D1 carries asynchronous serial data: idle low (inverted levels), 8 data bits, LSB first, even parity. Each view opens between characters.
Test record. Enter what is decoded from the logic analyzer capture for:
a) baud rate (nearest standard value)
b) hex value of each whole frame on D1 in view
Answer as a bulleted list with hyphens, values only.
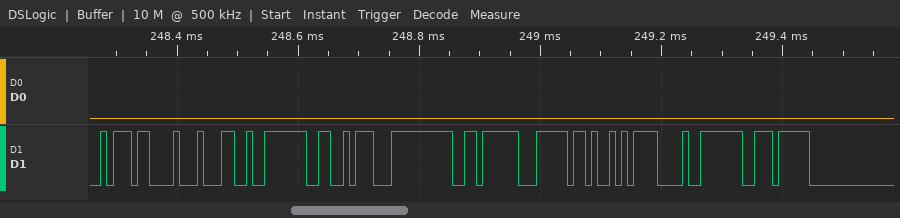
- 100000 baud
- 91, 77, 03, 16, 00, 02, 90, 85, 03, 04
